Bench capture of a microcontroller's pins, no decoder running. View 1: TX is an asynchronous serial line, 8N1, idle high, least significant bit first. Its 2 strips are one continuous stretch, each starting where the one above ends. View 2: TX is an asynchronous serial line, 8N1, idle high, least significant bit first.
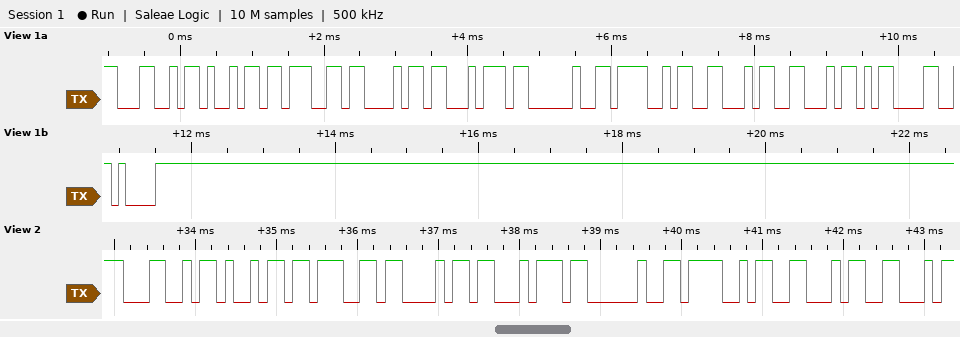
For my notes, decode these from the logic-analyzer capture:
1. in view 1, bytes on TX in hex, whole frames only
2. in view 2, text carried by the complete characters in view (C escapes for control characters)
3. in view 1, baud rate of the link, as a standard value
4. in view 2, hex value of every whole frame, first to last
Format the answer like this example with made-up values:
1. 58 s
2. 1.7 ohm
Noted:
1. 4C 69 67 68 74 20 4F 46 46 0D 0A
2. "Light OFF"
3. 9600 baud
4. 0x4C 0x69 0x67 0x68 0x74 0x20 0x4F 0x46 0x46
